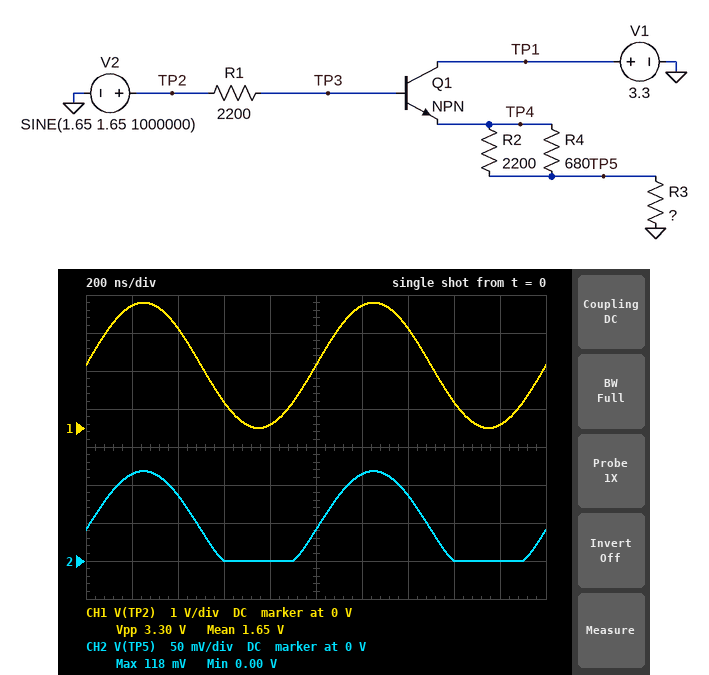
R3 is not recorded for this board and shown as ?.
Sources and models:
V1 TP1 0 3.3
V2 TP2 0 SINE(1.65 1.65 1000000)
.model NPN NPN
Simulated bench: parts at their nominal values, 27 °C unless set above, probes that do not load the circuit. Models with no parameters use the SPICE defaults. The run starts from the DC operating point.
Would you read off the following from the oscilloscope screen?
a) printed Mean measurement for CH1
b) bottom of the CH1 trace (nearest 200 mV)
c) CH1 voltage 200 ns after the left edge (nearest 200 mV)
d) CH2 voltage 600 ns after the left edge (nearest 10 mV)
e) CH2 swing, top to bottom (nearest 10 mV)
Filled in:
1.65 V
0 V
3.2 V
0 V
120 mV
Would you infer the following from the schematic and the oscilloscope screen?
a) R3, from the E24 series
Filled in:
27 Ω
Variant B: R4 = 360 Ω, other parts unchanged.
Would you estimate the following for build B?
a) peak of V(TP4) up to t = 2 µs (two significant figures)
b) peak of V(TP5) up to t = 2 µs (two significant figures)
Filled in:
2.3 V
190 mV
